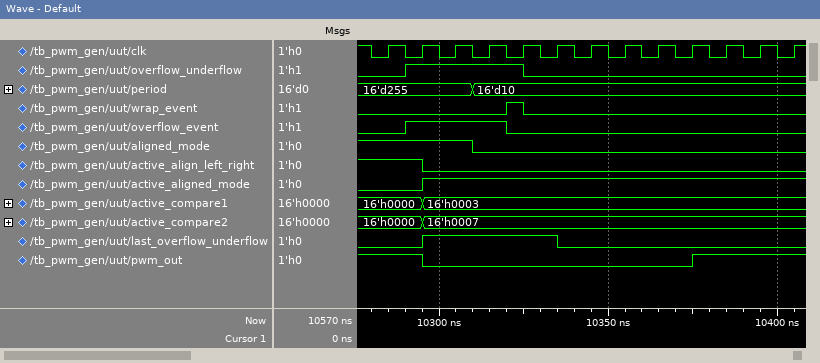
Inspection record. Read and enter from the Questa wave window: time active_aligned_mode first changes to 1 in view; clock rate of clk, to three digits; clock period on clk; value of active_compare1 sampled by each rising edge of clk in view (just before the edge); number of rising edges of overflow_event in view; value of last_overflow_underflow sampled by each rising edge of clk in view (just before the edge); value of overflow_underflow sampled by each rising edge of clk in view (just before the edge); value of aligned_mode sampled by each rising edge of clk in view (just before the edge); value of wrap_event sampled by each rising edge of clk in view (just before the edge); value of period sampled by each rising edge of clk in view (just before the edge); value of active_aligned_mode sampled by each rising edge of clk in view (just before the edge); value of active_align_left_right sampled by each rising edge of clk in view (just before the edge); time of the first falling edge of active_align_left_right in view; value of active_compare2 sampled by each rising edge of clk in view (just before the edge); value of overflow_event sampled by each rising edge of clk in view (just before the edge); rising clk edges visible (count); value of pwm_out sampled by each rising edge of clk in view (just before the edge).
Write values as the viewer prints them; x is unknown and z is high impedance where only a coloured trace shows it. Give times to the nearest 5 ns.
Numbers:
10295 ns
100 MHz
10 ns
16'h0000, 16'h0000, 16'h0003, 16'h0003, 16'h0003, 16'h0003, 16'h0003, 16'h0003, 16'h0003, 16'h0003, 16'h0003, 16'h0003, 16'h0003
1
0 0 1 1 1 1 0 0 0 0 0 0 0
0 1 1 1 1 0 0 0 0 0 0 0 0
1 1 1 0 0 0 0 0 0 0 0 0 0
0 0 0 0 1 0 0 0 0 0 0 0 0
16'd255, 16'd255, 16'd255, 16'd10, 16'd10, 16'd10, 16'd10, 16'd10, 16'd10, 16'd10, 16'd10, 16'd10, 16'd10
0 0 1 1 1 1 1 1 1 1 1 1 1
1 1 0 0 0 0 0 0 0 0 0 0 0
10295 ns
16'h0000, 16'h0000, 16'h0007, 16'h0007, 16'h0007, 16'h0007, 16'h0007, 16'h0007, 16'h0007, 16'h0007, 16'h0007, 16'h0007, 16'h0007
0 1 1 1 0 0 0 0 0 0 0 0 0
13
1 1 0 0 0 0 0 0 0 0 1 1 1
